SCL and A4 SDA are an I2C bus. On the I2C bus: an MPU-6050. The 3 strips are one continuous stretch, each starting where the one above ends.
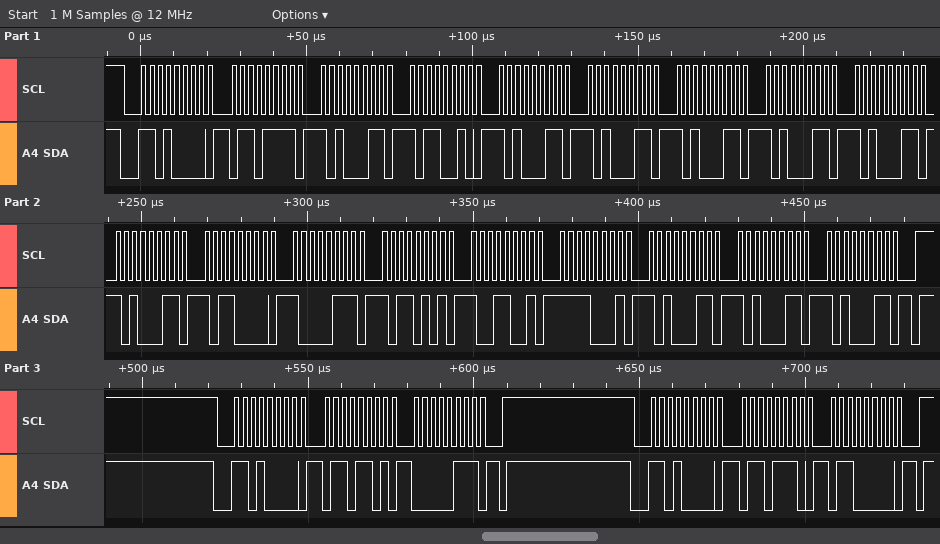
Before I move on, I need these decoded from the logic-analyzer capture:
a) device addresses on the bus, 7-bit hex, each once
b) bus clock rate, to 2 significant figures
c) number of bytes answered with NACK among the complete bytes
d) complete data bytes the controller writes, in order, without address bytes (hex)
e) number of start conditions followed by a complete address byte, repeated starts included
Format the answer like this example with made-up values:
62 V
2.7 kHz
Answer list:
0x68
400 kHz
0
6F A3 B2 A3 A3 A3 A3 A3 A3 B0 87 B5 99 F1 A3 A3 A3 6D 07 6E 60
3
